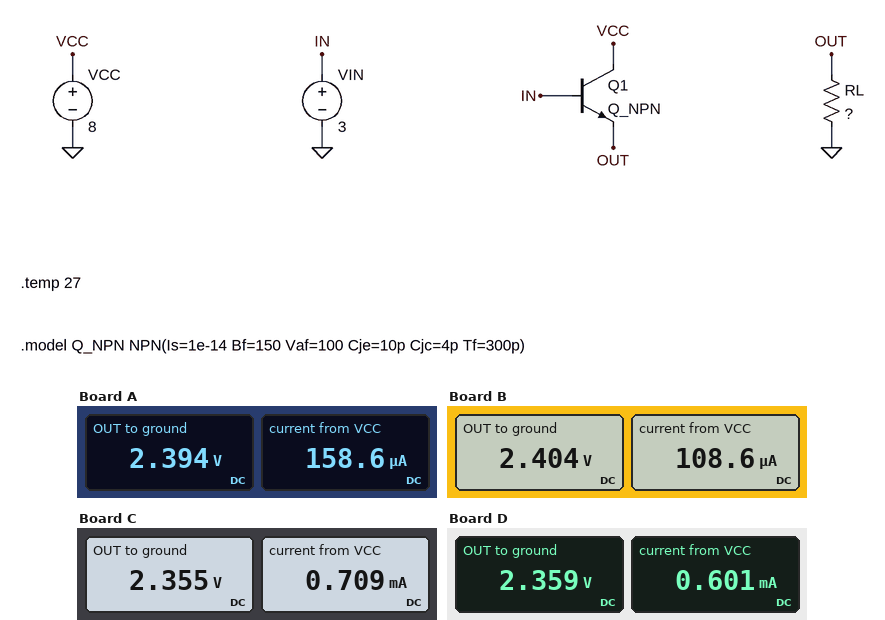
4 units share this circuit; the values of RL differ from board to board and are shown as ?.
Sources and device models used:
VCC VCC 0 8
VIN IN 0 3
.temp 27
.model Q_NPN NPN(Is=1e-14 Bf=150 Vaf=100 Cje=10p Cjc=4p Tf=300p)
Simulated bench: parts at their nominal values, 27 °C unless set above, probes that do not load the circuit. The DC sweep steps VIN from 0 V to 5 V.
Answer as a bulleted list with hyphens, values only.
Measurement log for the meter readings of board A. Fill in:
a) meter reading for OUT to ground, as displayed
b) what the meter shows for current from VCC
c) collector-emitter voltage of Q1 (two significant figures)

- 2.394 V
- 158.6 µA
- 5.6 V
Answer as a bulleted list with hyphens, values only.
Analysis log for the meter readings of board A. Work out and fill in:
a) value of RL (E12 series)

- 15 kΩ
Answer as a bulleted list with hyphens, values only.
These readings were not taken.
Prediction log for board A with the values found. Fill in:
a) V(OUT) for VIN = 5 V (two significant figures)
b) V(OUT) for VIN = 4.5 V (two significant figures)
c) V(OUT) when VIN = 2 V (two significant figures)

- 4.4 V
- 3.9 V
- 1.4 V
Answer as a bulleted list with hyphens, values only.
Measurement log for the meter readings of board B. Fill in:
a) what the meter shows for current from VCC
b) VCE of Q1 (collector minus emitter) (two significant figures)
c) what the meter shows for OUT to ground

- 108.6 µA
- 5.6 V
- 2.404 V
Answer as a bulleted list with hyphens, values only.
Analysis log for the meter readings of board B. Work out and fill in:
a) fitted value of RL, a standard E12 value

- 22 kΩ
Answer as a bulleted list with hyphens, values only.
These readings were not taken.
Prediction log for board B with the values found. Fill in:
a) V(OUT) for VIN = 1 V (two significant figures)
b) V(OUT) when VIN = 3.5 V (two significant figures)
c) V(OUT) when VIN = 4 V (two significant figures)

- 450 mV
- 2.9 V
- 3.4 V
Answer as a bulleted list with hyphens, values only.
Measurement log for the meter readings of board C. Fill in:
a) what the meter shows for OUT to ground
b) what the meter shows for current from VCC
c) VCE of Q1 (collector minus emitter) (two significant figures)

- 2.355 V
- 0.709 mA
- 5.6 V
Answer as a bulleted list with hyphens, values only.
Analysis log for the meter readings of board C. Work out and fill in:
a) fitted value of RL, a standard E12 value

- 3.3 kΩ
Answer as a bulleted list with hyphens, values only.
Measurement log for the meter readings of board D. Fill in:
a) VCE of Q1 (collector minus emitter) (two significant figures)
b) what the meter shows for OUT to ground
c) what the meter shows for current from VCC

- 5.6 V
- 2.359 V
- 0.601 mA
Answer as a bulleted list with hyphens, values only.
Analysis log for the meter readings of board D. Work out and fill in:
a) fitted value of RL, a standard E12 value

- 3.9 kΩ
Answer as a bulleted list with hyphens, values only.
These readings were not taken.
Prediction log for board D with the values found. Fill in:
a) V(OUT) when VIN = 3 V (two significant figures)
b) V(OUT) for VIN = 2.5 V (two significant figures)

- 2.4 V
- 1.9 V
